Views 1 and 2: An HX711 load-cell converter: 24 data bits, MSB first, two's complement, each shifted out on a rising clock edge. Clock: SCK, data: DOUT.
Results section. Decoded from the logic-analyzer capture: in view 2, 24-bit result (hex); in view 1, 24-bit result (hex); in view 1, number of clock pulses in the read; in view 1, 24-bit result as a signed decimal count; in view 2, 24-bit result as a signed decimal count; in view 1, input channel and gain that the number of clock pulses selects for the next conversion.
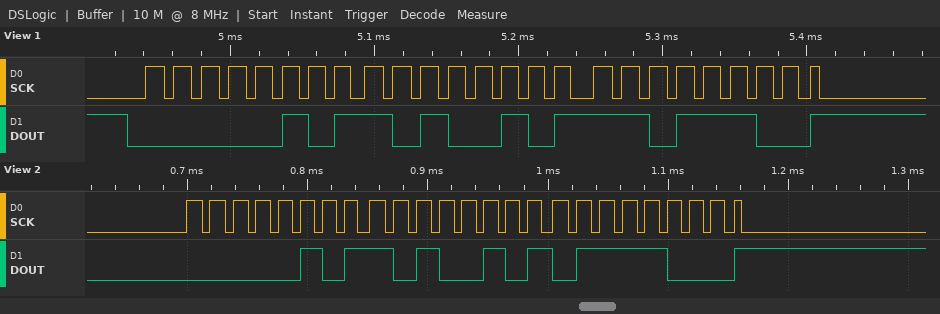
0x05A578
0x05A5DC
25
370140
370040
channel A, gain 128
